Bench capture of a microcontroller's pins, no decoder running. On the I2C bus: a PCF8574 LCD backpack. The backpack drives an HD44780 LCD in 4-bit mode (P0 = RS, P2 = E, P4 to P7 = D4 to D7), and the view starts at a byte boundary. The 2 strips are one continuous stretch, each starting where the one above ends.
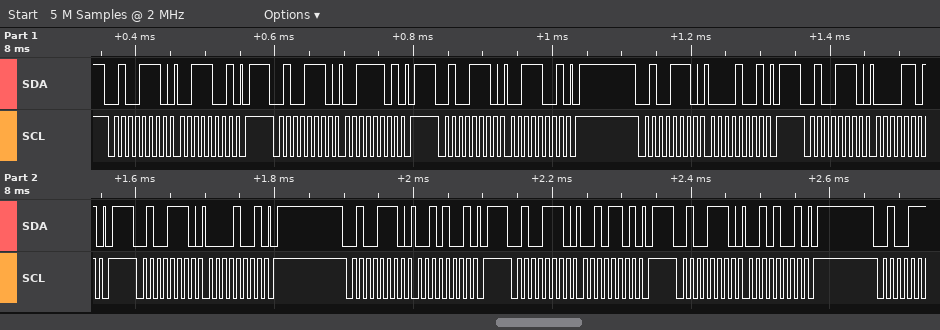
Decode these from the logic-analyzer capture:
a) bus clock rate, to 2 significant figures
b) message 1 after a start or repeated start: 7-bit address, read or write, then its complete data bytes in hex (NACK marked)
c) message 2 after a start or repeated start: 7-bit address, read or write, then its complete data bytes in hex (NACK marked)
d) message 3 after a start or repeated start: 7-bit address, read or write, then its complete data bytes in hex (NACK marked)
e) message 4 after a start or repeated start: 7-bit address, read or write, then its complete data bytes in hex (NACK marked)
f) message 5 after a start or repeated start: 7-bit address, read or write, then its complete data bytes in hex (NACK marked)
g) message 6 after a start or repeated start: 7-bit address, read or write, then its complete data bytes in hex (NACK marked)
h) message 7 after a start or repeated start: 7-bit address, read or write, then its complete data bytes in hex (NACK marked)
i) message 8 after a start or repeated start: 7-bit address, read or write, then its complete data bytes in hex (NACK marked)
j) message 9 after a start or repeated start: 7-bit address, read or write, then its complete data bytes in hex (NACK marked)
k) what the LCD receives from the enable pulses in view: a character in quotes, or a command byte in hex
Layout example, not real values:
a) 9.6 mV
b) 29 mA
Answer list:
a) 100 kHz
b) 0x27 write: 39
c) 0x27 write: 3D
d) 0x27 write: 39
e) 0x27 write: 09
f) 0x27 write: 0D
g) 0x27 write: 09
h) 0x27 write: 29
i) 0x27 write: 2D
j) 0x27 write: 29
k) '0'
